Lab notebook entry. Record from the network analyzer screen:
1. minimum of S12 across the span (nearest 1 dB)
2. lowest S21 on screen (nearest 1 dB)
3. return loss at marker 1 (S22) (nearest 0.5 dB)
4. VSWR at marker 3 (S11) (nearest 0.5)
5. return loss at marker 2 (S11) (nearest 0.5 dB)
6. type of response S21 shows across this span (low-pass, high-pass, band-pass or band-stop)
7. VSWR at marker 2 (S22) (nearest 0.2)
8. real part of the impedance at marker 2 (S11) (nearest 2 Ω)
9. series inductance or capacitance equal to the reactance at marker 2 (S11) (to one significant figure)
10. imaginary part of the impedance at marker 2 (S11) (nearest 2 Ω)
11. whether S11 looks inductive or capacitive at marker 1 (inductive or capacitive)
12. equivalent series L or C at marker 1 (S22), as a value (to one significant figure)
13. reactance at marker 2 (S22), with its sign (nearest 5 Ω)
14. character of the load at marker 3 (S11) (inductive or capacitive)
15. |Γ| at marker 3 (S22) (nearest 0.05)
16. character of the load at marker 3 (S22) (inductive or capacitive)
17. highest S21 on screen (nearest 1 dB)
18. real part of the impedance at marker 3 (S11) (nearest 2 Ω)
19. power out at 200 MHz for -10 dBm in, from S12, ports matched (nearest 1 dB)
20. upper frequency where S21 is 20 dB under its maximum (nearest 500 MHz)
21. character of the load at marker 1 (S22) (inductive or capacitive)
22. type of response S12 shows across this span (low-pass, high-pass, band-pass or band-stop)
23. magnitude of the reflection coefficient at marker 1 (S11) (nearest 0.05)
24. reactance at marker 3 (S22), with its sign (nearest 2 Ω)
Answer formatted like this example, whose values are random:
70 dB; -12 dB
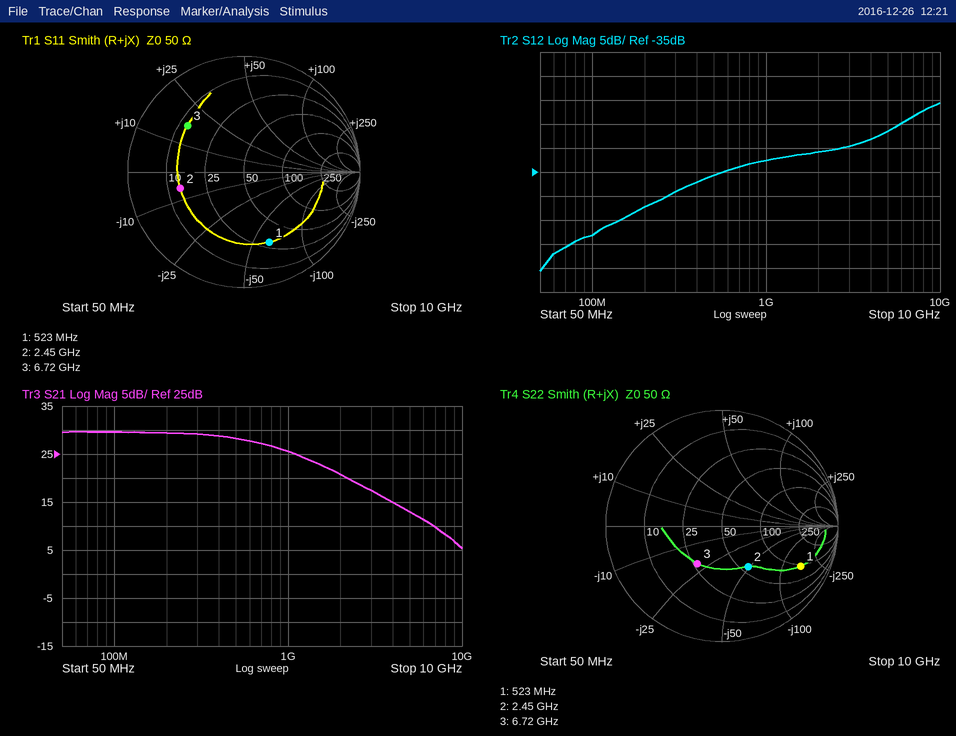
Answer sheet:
-56 dB; 5 dB; 2.5 dB; 4.5; 5.0 dB; low-pass; 2.4; 14 Ω; 10 pF; -6 Ω; capacitive; 2 pF; -50 Ω; inductive; 0.40; capacitive; 30 dB; 12 Ω; -52 dBm; 7.0 GHz; capacitive; high-pass; 0.65; -20 Ω
